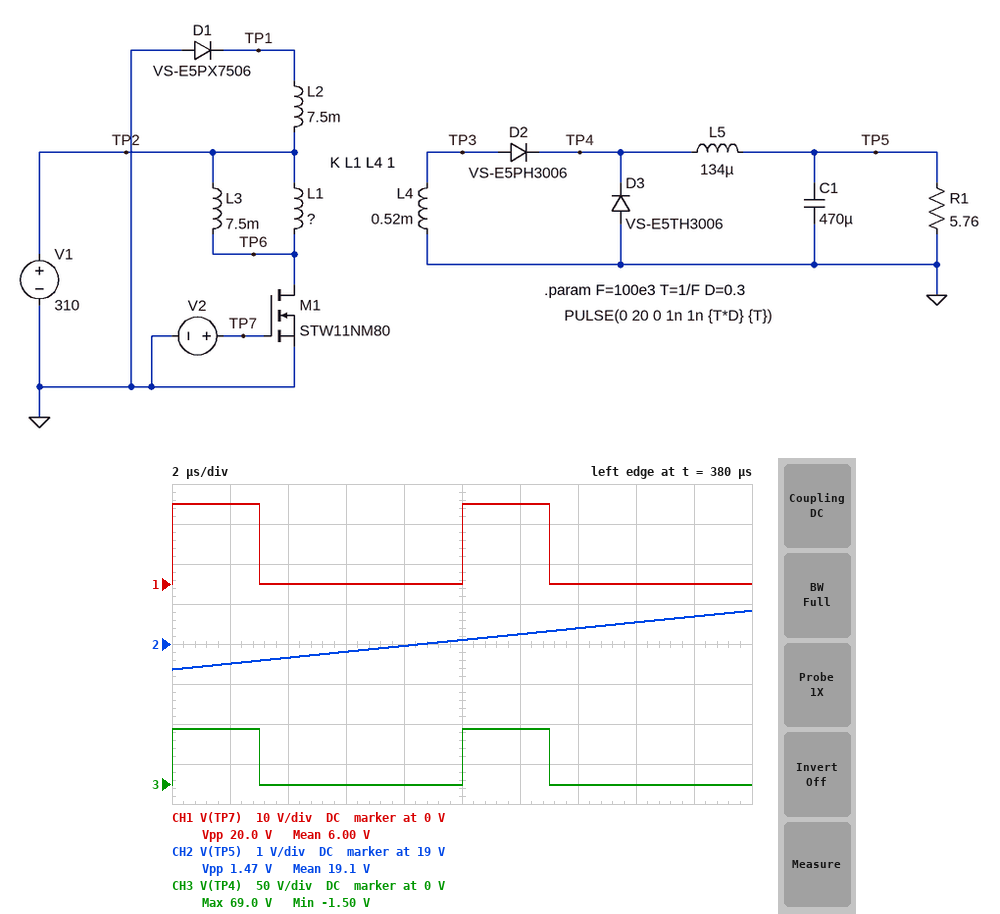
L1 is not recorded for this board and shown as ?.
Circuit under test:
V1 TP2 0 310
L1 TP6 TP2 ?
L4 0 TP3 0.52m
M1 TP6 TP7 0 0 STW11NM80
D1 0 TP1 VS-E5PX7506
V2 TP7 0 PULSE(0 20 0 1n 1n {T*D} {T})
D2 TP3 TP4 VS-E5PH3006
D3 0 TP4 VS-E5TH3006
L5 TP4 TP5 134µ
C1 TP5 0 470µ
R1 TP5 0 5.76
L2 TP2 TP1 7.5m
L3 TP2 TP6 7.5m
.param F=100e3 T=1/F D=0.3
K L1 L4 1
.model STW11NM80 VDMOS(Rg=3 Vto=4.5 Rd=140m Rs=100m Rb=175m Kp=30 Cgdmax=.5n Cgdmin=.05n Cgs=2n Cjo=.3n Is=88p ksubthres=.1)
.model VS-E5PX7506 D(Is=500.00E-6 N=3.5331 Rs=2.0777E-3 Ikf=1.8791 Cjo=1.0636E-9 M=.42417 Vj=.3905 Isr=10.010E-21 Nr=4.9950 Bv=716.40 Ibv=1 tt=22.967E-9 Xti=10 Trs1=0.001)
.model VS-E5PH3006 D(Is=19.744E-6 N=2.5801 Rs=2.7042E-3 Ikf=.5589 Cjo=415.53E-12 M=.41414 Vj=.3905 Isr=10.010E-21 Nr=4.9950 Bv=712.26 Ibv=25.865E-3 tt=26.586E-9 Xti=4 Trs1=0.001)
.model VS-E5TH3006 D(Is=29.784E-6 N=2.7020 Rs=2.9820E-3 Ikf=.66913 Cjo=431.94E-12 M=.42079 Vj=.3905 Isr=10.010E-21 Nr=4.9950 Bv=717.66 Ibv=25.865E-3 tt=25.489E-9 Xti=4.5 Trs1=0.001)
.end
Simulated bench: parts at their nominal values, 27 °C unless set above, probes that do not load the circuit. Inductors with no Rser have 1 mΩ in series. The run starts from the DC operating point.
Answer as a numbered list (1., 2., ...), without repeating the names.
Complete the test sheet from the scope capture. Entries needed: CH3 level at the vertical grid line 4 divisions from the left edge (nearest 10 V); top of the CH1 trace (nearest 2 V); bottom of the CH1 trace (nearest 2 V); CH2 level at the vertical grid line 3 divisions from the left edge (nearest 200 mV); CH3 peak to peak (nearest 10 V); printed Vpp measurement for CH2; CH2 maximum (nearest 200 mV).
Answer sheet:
1. 0 V
2. 20 V
3. 0 V
4. 18.8 V
5. 70 V
6. 1.47 V
7. 19.8 V
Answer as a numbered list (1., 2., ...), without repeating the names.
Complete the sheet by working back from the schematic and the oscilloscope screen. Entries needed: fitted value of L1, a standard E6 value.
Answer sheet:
1. 10 mH
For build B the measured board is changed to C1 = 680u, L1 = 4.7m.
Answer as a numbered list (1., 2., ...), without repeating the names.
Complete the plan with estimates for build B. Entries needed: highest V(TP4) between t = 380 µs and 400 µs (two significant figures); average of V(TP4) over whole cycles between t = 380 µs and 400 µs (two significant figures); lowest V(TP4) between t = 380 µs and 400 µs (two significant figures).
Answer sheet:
1. 100 V
2. 29 V
3. -1.5 V
